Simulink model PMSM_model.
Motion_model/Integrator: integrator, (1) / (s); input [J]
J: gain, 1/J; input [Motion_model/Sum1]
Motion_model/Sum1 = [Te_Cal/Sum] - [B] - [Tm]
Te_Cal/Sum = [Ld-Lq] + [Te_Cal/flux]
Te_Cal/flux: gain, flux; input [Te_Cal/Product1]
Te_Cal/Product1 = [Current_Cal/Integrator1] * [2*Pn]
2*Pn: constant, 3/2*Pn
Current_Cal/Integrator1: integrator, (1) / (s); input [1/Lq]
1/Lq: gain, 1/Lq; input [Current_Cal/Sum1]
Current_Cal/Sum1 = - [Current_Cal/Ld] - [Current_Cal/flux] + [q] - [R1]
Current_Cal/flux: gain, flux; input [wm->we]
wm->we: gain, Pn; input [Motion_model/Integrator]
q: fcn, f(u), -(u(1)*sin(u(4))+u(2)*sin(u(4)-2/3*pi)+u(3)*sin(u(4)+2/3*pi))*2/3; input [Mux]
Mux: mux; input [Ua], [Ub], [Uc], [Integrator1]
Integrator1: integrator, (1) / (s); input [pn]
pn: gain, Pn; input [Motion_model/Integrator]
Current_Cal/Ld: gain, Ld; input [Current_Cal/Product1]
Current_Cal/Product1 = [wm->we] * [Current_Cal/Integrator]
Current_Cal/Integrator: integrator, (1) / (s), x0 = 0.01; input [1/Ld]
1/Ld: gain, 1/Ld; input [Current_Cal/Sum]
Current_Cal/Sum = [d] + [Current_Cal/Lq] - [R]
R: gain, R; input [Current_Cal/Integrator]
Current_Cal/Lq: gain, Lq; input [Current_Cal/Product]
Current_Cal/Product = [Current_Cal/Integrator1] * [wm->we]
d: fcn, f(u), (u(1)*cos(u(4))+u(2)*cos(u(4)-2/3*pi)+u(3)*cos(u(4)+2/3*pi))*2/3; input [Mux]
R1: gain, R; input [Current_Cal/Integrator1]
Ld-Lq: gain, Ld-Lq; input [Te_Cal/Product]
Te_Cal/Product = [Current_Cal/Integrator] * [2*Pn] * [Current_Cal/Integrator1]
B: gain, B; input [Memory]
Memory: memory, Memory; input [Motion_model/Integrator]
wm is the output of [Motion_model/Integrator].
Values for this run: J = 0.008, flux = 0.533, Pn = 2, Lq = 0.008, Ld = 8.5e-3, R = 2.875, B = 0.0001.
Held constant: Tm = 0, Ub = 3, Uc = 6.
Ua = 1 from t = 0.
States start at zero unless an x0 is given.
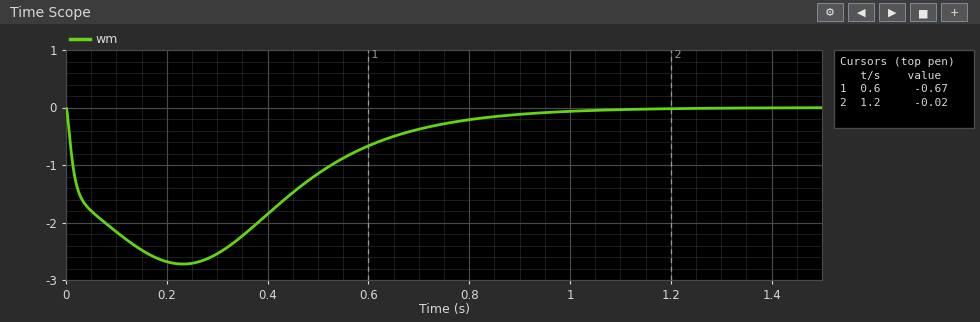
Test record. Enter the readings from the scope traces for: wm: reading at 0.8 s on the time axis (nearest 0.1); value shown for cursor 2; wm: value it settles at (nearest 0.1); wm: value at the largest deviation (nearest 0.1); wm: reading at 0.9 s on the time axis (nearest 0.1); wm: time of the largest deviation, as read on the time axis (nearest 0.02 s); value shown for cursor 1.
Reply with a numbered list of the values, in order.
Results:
1. -0.2
2. -0.02
3. 0.0
4. -2.7
5. -0.1
6. 0.24 s
7. -0.67
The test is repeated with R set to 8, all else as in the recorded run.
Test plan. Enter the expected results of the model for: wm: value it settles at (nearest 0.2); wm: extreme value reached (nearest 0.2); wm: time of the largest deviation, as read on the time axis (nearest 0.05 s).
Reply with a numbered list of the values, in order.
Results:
1. 0.0
2. -2.6
3. 0.30 s
